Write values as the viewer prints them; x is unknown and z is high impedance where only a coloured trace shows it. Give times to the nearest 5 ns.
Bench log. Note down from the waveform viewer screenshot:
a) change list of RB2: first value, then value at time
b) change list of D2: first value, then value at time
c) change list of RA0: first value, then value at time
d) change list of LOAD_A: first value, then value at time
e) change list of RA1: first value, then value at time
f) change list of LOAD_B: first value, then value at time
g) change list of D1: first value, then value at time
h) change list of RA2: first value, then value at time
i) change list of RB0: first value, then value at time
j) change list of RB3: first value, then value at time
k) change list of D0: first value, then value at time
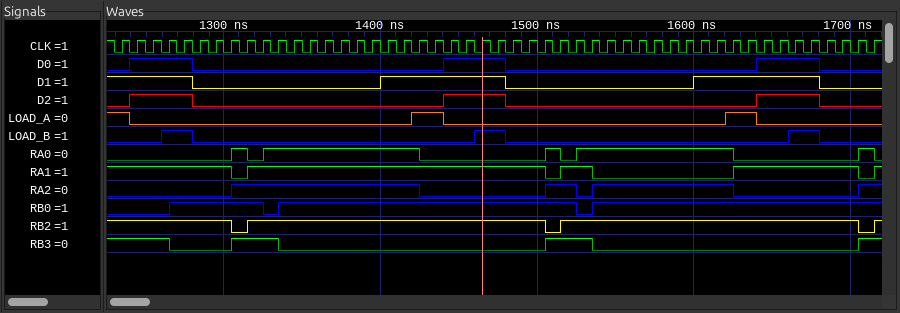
1, 0 at 1305 ns, 1 at 1315 ns, 0 at 1505 ns, 1 at 1515 ns, 0 at 1705 ns, 1 at 1715 ns
0, 1 at 1240 ns, 0 at 1280 ns, 1 at 1440 ns, 0 at 1480 ns, 1 at 1640 ns, 0 at 1680 ns
0, 1 at 1305 ns, 0 at 1315 ns, 1 at 1325 ns, 0 at 1425 ns, 1 at 1505 ns, 0 at 1515 ns, 1 at 1525 ns, 0 at 1625 ns, 1 at 1705 ns, 0 at 1715 ns
1, 0 at 1240 ns, 1 at 1420 ns, 0 at 1440 ns, 1 at 1620 ns, 0 at 1640 ns
1, 0 at 1305 ns, 1 at 1315 ns, 0 at 1505 ns, 1 at 1515 ns, 0 at 1535 ns, 1 at 1625 ns, 0 at 1705 ns, 1 at 1715 ns
0, 1 at 1260 ns, 0 at 1280 ns, 1 at 1460 ns, 0 at 1480 ns, 1 at 1660 ns, 0 at 1680 ns
1, 0 at 1280 ns, 1 at 1400 ns, 0 at 1480 ns, 1 at 1600 ns, 0 at 1680 ns
0, 1 at 1305 ns, 0 at 1425 ns, 1 at 1505 ns, 0 at 1525 ns, 1 at 1535 ns, 0 at 1625 ns, 1 at 1705 ns
0, 1 at 1265 ns, 0 at 1325 ns, 1 at 1335 ns, 0 at 1525 ns, 1 at 1535 ns
1, 0 at 1265 ns, 1 at 1305 ns, 0 at 1335 ns, 1 at 1505 ns, 0 at 1535 ns, 1 at 1705 ns
0, 1 at 1240 ns, 0 at 1280 ns, 1 at 1440 ns, 0 at 1480 ns, 1 at 1640 ns, 0 at 1680 ns
